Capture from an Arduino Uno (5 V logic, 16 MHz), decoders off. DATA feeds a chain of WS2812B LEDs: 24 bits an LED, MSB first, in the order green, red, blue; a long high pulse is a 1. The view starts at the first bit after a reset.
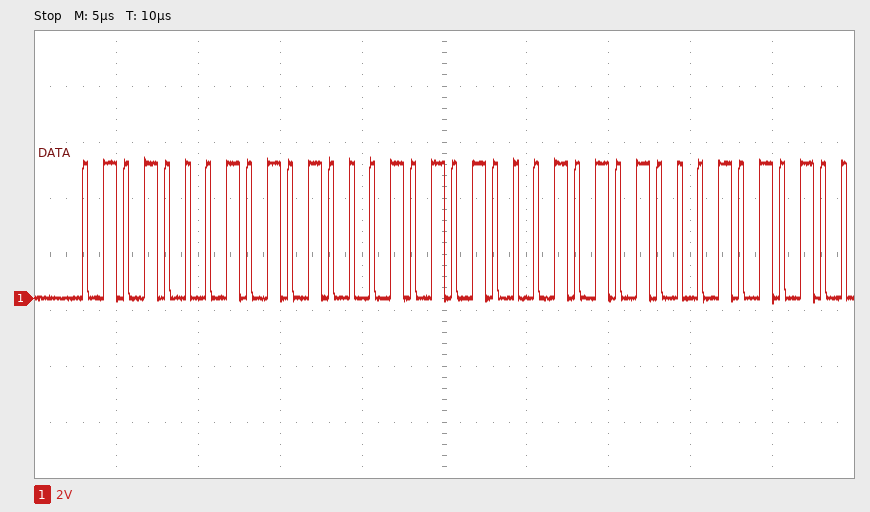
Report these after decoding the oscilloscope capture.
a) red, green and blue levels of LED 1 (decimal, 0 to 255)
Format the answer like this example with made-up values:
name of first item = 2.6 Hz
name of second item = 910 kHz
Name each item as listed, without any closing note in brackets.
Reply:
red, green and blue levels of LED 1 = 81, 81, 81
